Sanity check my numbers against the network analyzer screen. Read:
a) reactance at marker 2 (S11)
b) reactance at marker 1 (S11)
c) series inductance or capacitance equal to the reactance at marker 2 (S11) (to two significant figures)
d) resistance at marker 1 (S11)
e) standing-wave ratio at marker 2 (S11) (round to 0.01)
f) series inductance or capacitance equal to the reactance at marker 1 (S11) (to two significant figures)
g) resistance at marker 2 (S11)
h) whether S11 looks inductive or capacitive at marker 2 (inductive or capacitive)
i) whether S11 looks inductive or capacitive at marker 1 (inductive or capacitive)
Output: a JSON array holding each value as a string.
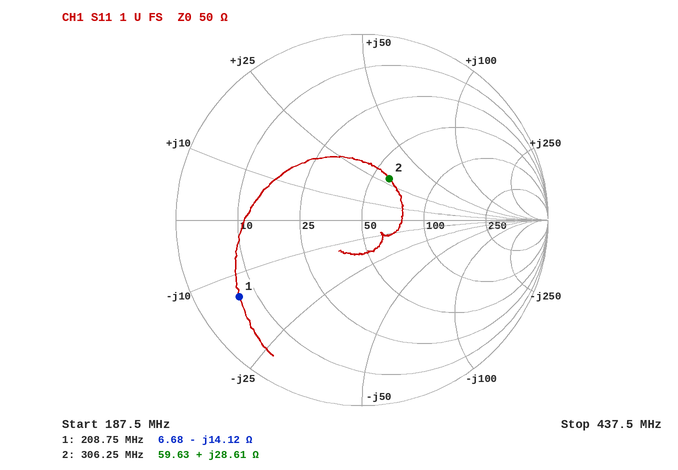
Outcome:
["+28.61 Ω", "-14.12 Ω", "15 nH", "6.68 Ω", "1.73", "54 pF", "59.63 Ω", "inductive", "capacitive"]
